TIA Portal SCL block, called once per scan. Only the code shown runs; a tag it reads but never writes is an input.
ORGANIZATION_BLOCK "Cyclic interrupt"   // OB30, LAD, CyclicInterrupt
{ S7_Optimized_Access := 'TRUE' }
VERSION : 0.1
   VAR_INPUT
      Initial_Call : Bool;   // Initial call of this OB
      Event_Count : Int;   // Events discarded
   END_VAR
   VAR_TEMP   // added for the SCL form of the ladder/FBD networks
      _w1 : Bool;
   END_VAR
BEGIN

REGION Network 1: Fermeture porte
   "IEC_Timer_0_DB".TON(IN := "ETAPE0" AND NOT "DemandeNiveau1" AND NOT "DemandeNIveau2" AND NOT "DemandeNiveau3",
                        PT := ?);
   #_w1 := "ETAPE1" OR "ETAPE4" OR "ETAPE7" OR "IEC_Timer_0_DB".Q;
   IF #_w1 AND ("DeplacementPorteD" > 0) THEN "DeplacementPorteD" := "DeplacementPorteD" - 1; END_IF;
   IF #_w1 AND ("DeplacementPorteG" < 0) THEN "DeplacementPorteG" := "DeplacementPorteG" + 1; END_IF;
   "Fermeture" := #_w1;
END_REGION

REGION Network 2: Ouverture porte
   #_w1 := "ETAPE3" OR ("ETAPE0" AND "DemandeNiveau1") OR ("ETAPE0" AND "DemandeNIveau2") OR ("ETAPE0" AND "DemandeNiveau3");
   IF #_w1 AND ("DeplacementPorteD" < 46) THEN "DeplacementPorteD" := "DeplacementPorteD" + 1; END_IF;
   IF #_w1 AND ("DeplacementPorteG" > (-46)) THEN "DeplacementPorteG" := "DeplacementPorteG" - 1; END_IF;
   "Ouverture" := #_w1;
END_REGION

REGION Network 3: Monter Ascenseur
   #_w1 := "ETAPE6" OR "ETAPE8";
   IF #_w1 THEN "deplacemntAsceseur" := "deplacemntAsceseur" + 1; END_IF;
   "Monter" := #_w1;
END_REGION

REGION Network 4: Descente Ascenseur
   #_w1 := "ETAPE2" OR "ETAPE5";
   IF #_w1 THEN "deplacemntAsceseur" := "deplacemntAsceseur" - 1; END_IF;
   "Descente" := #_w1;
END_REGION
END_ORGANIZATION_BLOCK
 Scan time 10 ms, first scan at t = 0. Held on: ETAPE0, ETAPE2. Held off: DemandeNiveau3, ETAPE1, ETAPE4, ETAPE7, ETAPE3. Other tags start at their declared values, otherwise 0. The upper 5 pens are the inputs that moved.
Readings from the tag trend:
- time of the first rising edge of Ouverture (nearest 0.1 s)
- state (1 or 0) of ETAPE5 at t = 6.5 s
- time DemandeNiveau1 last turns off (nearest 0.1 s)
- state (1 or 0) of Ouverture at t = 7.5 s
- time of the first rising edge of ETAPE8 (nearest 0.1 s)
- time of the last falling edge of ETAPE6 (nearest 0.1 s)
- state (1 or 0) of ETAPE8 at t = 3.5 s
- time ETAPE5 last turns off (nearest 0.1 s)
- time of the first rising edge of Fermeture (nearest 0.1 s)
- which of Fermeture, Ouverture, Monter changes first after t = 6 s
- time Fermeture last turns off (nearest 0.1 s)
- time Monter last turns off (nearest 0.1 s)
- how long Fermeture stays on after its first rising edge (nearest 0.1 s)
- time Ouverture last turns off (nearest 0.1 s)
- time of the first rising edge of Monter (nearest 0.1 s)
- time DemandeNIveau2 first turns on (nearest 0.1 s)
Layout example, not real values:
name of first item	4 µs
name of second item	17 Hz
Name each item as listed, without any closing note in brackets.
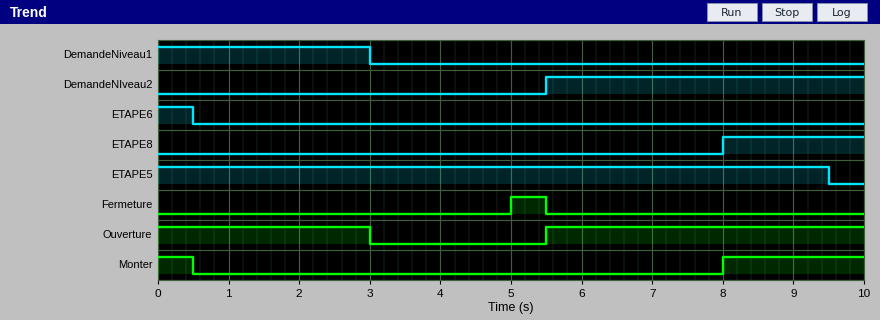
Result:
time of the first rising edge of Ouverture	5.5 s
state (1 or 0) of ETAPE5 at t = 6.5 s	1
time DemandeNiveau1 last turns off	3.0 s
state (1 or 0) of Ouverture at t = 7.5 s	1
time of the first rising edge of ETAPE8	8.0 s
time of the last falling edge of ETAPE6	0.5 s
state (1 or 0) of ETAPE8 at t = 3.5 s	0
time ETAPE5 last turns off	9.5 s
time of the first rising edge of Fermeture	5.0 s
which of Fermeture, Ouverture, Monter changes first after t = 6 s	Monter
time Fermeture last turns off	5.5 s
time Monter last turns off	0.5 s
how long Fermeture stays on after its first rising edge	0.5 s
time Ouverture last turns off	3.0 s
time of the first rising edge of Monter	8.0 s
time DemandeNIveau2 first turns on	5.5 s
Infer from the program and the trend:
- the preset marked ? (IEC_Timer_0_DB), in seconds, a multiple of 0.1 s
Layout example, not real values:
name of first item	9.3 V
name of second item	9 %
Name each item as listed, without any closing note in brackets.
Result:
the preset marked ? (IEC_Timer_0_DB), in seconds, a multiple of 0.1 s	2.0 s
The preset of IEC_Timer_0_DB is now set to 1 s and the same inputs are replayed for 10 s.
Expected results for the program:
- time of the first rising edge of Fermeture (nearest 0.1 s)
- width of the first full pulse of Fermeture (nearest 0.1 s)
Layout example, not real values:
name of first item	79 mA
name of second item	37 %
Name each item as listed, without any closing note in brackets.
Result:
time of the first rising edge of Fermeture	4.0 s
width of the first full pulse of Fermeture	1.5 s
